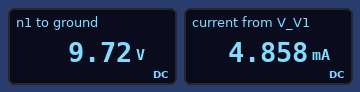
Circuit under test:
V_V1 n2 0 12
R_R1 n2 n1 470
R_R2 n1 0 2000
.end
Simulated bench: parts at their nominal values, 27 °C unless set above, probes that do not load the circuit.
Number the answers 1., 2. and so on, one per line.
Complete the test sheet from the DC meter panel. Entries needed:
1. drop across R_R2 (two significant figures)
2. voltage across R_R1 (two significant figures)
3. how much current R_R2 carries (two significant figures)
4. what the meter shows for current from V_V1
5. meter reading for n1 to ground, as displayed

1. 9.7 V
2. 2.3 V
3. 4.9 mA
4. 4.858 mA
5. 9.72 V
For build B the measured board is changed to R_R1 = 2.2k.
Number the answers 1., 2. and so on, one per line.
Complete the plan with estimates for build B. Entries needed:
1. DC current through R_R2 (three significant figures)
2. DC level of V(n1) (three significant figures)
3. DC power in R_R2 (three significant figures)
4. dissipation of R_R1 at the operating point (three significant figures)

1. 2.86 mA
2. 5.71 V
3. 16.3 mW
4. 18.0 mW
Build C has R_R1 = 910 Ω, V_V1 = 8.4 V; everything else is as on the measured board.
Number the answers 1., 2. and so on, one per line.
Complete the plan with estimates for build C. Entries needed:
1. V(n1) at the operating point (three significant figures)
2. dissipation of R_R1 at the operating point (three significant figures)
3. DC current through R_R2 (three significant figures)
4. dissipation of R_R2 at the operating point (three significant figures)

1. 5.77 V
2. 7.58 mW
3. 2.89 mA
4. 16.7 mW
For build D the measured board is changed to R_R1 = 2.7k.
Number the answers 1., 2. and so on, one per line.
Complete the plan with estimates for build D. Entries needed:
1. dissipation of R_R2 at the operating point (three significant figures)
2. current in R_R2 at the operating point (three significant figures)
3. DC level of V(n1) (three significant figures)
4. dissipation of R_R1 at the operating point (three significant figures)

1. 13.0 mW
2. 2.55 mA
3. 5.11 V
4. 17.6 mW
